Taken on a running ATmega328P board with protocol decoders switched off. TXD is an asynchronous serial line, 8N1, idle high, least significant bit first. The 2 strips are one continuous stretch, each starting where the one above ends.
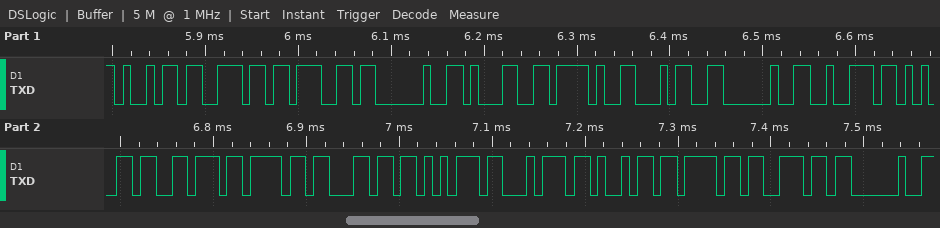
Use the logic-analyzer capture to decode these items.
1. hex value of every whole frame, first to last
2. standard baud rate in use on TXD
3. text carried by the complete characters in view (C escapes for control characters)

69 6E 67 20 31 2F 34 20 72 65 76 6F 6C 75 74 69 6F 6E 20
115200 baud
"ing 1/4 revolution "
